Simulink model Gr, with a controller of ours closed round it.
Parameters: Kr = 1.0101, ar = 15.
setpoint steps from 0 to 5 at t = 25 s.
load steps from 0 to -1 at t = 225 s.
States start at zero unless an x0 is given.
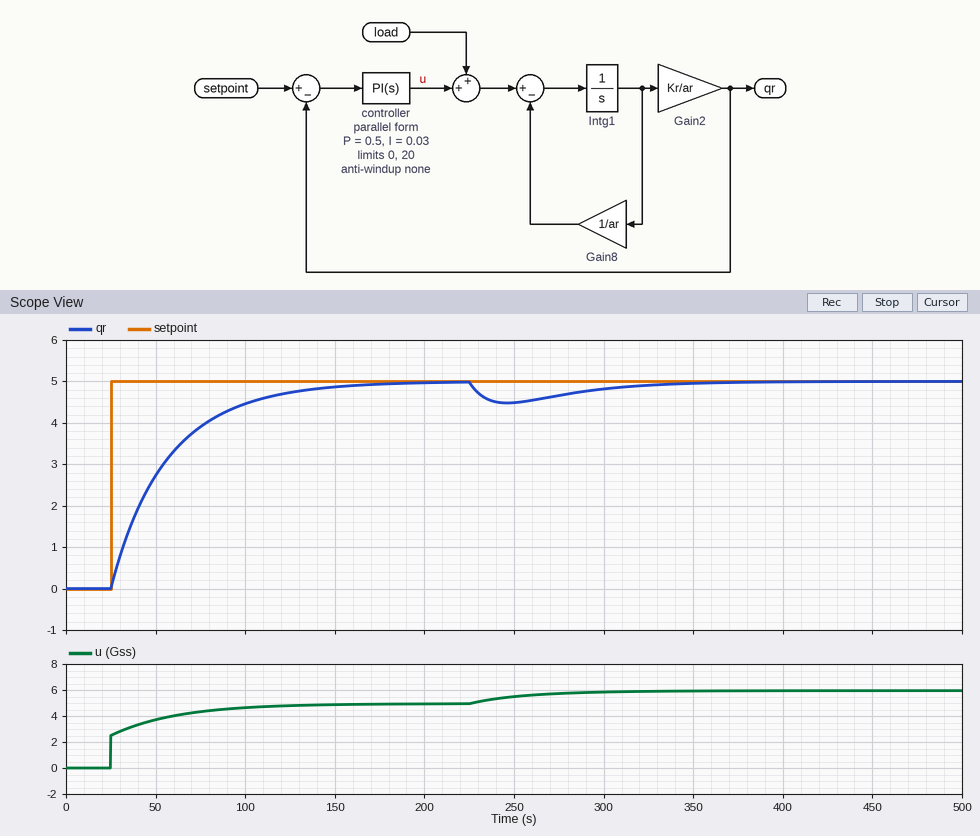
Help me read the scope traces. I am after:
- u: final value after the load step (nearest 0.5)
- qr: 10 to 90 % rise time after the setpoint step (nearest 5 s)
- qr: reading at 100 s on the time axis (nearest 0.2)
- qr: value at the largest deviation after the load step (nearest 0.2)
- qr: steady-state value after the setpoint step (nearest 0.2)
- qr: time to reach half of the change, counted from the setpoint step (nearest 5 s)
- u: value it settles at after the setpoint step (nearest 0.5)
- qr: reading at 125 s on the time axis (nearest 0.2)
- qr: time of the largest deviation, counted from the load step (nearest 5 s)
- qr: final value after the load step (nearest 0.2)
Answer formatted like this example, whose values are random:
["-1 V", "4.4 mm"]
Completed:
["6.0", "75 s", "4.4", "4.4", "5.0", "20 s", "5.0", "4.8", "20 s", "5.0"]
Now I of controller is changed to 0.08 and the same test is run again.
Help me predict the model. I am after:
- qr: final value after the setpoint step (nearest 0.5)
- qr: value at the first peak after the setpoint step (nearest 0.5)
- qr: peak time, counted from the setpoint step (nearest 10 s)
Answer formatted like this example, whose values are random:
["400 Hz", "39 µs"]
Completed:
["5.0", "5.5", "50 s"]
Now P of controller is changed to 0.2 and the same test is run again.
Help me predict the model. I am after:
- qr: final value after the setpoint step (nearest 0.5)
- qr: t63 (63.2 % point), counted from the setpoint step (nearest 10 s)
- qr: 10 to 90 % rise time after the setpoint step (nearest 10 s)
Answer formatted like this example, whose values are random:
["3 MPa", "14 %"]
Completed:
["5.0", "40 s", "60 s"]
